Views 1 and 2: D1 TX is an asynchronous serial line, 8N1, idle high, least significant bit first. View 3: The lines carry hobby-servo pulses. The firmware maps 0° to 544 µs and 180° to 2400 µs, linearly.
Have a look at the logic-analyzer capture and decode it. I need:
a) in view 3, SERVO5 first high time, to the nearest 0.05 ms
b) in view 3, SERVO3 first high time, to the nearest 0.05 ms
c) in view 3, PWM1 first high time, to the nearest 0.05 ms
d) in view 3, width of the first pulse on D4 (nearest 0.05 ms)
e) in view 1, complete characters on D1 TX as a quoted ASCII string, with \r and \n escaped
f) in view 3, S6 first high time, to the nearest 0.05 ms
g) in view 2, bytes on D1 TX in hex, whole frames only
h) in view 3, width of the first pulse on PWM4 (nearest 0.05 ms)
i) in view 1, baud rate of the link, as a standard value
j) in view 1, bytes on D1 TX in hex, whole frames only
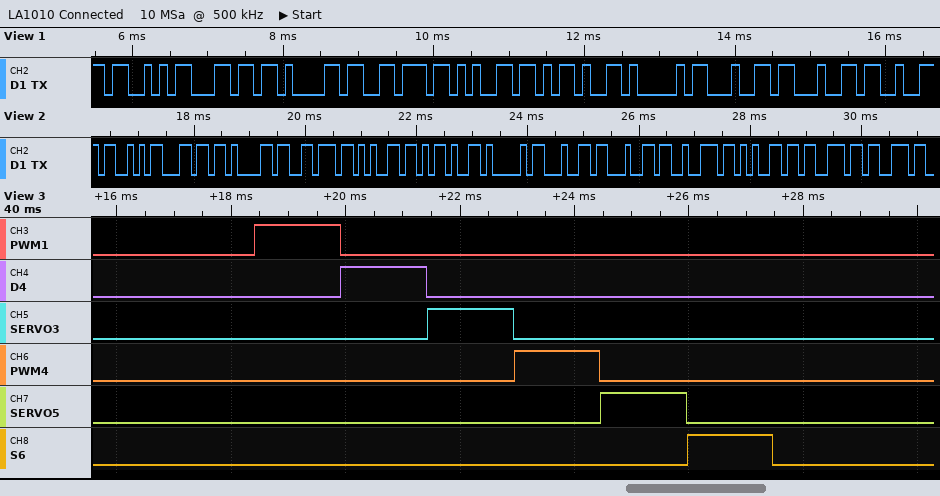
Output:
1.50 ms
1.50 ms
1.50 ms
1.50 ms
"Slave-Add"
1.50 ms
53 6C 61 76 65 2D 41 64 64 72 65 73 73
1.50 ms
9600 baud
53 6C 61 76 65 2D 41 64 64
